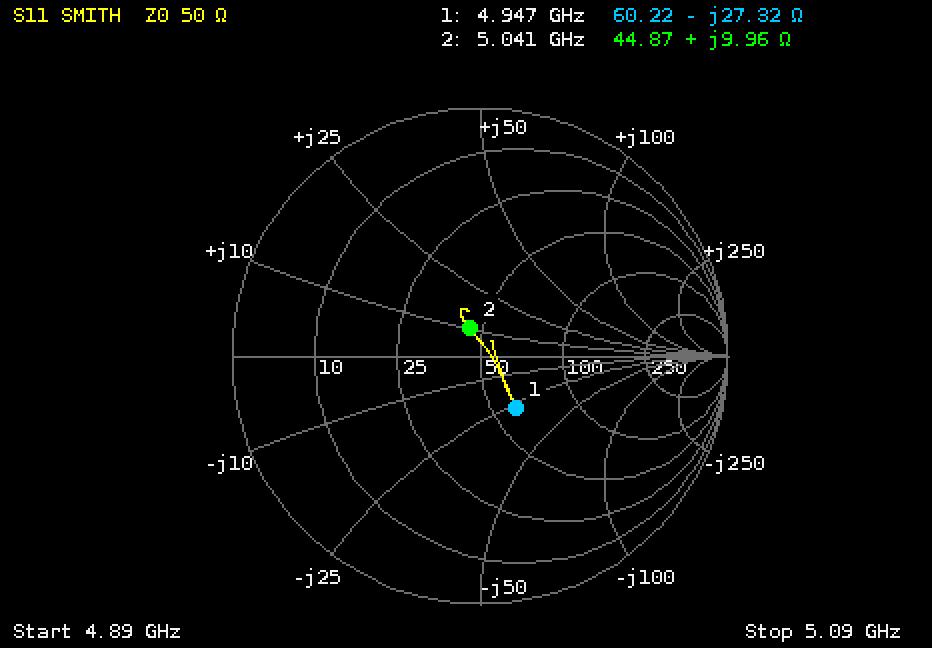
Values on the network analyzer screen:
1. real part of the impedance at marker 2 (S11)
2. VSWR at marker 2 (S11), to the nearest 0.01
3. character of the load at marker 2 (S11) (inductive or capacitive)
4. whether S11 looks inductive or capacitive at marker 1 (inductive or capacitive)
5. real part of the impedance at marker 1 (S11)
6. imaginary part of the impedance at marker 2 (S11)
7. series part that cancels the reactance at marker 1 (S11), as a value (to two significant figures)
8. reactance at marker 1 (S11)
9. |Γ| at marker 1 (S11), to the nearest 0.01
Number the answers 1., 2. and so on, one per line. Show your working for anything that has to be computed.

1. 44.87 Ω
2. 1.27
3. inductive
4. capacitive
5. 60.22 Ω
6. +9.96 Ω
7. L = 27.32 Ω/(2π × 4.947 GHz) ≈ 879 pH, so 880 pH to two significant figures
8. -27.32 Ω
9. 0.26
